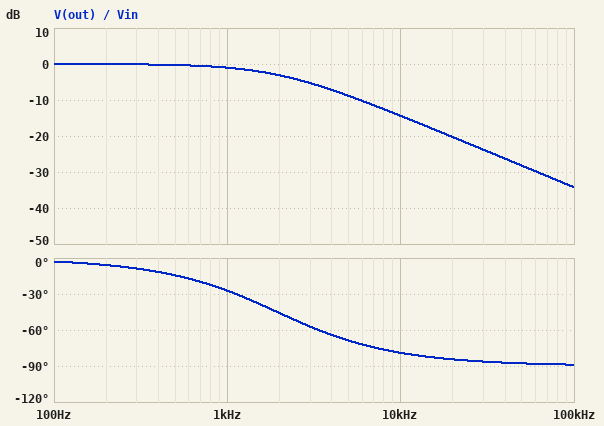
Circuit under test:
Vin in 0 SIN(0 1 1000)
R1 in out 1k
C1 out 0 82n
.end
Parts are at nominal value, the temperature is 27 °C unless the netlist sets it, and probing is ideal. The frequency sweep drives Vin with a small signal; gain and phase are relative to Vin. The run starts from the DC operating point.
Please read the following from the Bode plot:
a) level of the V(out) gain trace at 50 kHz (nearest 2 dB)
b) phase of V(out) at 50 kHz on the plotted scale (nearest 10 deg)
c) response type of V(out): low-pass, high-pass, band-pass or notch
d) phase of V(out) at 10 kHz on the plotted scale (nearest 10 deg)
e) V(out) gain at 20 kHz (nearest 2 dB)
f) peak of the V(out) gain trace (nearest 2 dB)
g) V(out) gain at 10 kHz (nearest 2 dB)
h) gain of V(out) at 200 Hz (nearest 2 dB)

-28 dB
-90 deg
low-pass
-80 deg
-20 dB
0 dB
-14 dB
0 dB
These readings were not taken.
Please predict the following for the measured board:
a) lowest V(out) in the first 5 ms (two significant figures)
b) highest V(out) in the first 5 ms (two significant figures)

-890 mV
900 mV
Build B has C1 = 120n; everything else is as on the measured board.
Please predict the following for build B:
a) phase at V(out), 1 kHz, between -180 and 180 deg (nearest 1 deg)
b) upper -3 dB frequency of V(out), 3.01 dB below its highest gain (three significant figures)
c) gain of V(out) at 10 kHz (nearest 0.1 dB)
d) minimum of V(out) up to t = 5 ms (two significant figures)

-37 deg
1.33 kHz
-17.6 dB
-800 mV
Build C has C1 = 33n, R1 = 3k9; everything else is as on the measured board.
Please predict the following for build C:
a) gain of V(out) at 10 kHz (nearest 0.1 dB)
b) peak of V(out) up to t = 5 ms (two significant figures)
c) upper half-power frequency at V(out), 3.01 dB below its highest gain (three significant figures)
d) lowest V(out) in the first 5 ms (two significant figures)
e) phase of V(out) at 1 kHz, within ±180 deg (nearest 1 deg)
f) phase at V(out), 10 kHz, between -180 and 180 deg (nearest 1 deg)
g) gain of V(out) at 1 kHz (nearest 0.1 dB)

-18.2 dB
810 mV
1.24 kHz
-780 mV
-39 deg
-83 deg
-2.2 dB
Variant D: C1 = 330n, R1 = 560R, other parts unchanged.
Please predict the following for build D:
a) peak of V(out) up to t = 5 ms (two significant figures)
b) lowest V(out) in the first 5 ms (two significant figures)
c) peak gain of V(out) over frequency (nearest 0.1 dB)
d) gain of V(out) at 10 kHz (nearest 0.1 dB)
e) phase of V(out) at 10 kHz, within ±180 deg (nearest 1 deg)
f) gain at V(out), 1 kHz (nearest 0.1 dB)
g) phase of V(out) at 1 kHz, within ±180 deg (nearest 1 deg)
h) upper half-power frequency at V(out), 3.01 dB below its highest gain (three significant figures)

720 mV
-650 mV
0 dB
-21.3 dB
-85 deg
-3.7 dB
-49 deg
861 Hz
